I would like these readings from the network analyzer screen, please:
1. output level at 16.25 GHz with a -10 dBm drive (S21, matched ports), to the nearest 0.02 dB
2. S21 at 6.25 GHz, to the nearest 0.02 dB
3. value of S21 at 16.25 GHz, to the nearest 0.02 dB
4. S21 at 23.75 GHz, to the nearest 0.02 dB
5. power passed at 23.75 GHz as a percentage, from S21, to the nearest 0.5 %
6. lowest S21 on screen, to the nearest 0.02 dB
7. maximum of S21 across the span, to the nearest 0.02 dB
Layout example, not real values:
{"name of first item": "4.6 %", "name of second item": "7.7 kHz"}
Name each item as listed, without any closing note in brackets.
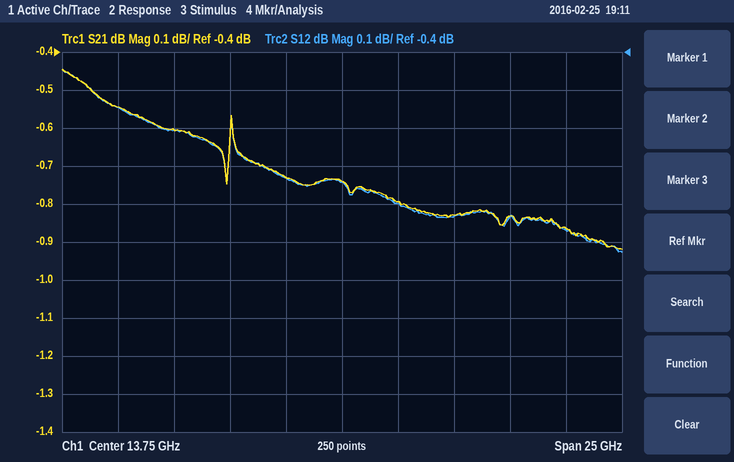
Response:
{"output level at 16.25 GHz with a -10 dBm drive (S21, matched ports), to the nearest 0.02 dB": "-10.80 dBm", "S21 at 6.25 GHz, to the nearest 0.02 dB": "-0.60 dB", "value of S21 at 16.25 GHz, to the nearest 0.02 dB": "-0.80 dB", "S21 at 23.75 GHz, to the nearest 0.02 dB": "-0.86 dB", "power passed at 23.75 GHz as a percentage, from S21, to the nearest 0.5 %": "82.0 %", "lowest S21 on screen, to the nearest 0.02 dB": "-0.92 dB", "maximum of S21 across the span, to the nearest 0.02 dB": "-0.44 dB"}
